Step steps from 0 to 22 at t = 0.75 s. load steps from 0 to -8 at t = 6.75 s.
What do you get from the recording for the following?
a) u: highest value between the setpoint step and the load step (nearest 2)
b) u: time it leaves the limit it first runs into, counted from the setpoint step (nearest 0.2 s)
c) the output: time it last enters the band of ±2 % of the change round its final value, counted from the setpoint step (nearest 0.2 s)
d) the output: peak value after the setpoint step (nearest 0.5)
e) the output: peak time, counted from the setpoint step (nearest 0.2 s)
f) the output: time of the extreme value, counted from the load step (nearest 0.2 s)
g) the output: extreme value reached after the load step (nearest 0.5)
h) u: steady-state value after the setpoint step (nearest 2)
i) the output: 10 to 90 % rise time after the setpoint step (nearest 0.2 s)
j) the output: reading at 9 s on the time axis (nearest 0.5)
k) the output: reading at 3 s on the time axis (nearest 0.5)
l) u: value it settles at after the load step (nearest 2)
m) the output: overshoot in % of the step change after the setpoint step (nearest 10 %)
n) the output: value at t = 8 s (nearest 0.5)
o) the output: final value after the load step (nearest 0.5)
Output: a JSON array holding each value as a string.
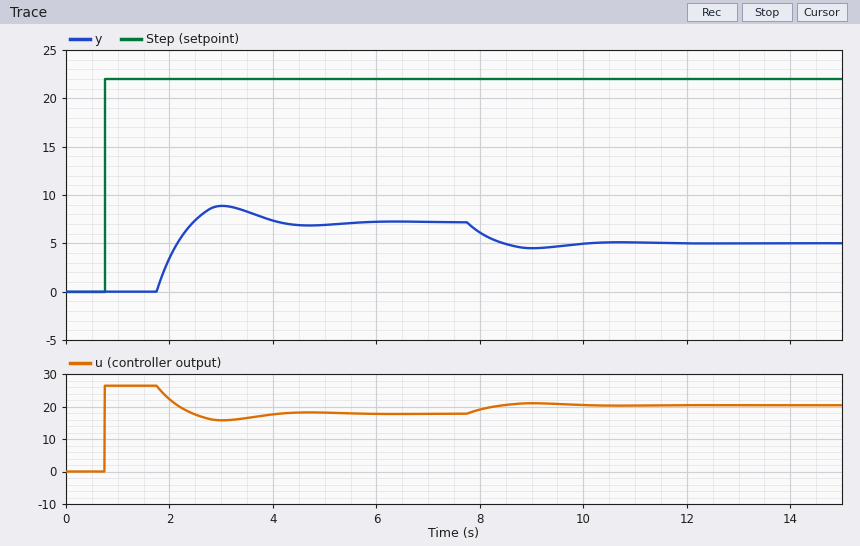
["26", "1.0 s", "4.6 s", "9.0", "2.2 s", "2.2 s", "4.5", "18", "0.6 s", "4.5", "9.0", "20", "20 %", "6.0", "5.0"]
